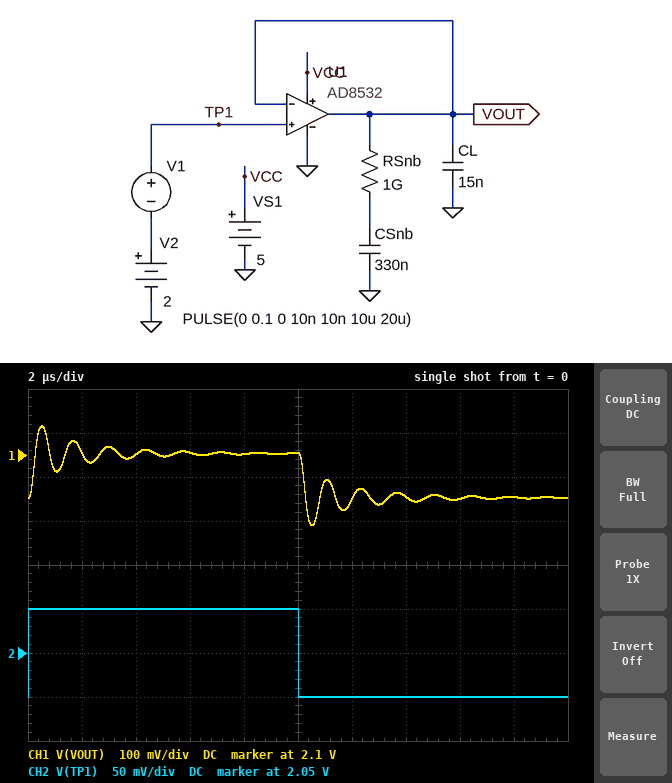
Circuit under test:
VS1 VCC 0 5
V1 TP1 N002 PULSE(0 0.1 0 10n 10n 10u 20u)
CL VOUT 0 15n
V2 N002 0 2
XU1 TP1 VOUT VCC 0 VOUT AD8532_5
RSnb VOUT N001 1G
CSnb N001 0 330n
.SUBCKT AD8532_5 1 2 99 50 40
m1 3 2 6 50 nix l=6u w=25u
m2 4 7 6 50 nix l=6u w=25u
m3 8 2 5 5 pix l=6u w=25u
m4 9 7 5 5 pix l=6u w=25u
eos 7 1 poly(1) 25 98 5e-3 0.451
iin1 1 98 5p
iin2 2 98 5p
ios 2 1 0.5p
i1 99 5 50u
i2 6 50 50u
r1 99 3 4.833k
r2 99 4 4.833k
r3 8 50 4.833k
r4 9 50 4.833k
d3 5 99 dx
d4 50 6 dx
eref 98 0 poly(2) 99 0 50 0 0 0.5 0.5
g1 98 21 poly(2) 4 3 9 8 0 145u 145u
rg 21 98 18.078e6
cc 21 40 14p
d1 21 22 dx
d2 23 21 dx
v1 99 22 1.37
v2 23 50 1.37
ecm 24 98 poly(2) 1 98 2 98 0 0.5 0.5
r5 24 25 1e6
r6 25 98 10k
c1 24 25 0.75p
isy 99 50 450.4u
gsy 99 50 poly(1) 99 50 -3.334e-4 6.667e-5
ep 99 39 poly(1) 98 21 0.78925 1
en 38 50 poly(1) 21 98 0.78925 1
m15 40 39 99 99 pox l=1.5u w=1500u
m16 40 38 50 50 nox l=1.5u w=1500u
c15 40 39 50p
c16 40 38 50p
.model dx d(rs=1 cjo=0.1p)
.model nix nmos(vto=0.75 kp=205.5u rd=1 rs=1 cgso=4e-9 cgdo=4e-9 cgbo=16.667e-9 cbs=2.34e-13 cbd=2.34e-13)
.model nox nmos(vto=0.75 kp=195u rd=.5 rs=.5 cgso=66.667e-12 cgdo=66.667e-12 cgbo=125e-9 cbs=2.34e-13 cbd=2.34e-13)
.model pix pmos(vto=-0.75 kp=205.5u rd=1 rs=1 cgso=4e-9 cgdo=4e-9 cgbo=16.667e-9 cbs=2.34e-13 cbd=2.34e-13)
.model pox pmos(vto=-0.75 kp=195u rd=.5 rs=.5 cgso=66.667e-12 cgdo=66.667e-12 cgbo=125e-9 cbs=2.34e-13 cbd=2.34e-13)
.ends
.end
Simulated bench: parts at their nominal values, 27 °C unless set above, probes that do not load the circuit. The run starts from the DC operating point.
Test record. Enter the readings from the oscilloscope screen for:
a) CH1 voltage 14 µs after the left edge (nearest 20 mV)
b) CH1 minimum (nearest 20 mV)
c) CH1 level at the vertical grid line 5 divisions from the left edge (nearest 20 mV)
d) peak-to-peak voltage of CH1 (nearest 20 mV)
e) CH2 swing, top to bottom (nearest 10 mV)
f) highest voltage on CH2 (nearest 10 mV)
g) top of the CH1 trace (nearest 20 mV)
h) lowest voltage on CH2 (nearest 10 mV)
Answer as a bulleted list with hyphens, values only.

- 2.00 V
- 1.94 V
- 2.10 V
- 220 mV
- 100 mV
- 2.10 V
- 2.16 V
- 2.00 V
